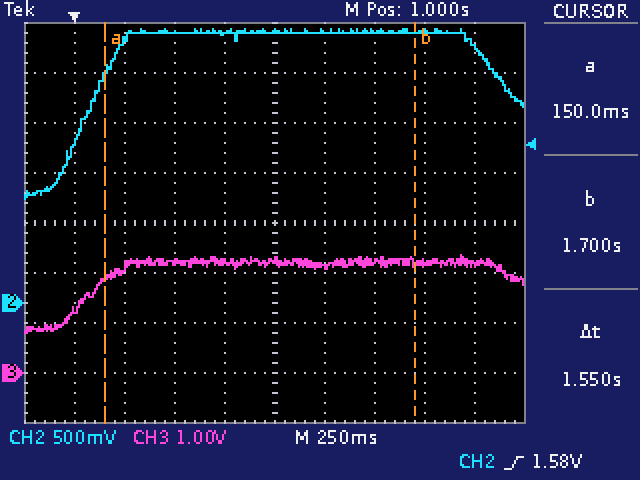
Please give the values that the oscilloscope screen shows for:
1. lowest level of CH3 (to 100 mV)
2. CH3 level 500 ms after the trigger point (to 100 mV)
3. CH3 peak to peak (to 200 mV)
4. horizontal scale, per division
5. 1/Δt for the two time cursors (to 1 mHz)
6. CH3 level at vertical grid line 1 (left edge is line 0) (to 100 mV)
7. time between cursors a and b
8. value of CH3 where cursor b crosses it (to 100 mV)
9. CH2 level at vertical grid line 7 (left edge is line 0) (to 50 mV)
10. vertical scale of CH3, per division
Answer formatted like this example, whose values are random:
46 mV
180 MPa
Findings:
800 mV
2.2 V
1.6 V
250 ms
645 mHz
1.2 V
1.55 s
2.2 V
2.70 V
1 V
